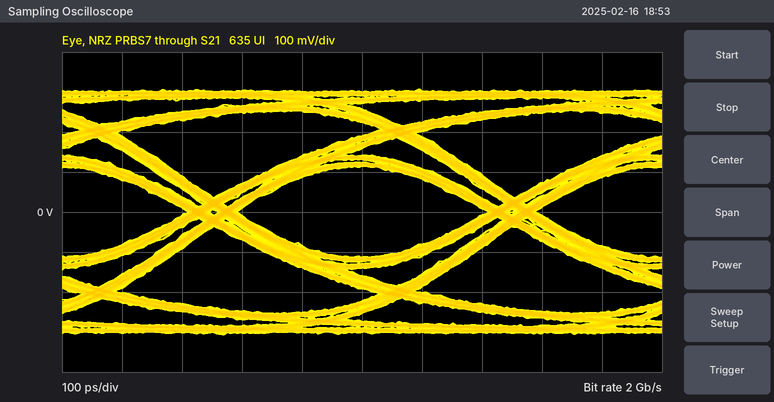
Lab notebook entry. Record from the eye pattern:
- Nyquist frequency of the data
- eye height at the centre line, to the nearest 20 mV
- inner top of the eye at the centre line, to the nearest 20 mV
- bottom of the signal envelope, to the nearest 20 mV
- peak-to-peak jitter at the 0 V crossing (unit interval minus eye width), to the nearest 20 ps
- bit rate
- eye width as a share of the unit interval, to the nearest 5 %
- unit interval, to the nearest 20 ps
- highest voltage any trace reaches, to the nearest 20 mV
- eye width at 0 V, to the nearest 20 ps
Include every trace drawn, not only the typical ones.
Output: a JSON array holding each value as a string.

["1 GHz", "220 mV", "120 mV", "-300 mV", "80 ps", "2 Gb/s", "85 %", "500 ps", "300 mV", "420 ps"]
